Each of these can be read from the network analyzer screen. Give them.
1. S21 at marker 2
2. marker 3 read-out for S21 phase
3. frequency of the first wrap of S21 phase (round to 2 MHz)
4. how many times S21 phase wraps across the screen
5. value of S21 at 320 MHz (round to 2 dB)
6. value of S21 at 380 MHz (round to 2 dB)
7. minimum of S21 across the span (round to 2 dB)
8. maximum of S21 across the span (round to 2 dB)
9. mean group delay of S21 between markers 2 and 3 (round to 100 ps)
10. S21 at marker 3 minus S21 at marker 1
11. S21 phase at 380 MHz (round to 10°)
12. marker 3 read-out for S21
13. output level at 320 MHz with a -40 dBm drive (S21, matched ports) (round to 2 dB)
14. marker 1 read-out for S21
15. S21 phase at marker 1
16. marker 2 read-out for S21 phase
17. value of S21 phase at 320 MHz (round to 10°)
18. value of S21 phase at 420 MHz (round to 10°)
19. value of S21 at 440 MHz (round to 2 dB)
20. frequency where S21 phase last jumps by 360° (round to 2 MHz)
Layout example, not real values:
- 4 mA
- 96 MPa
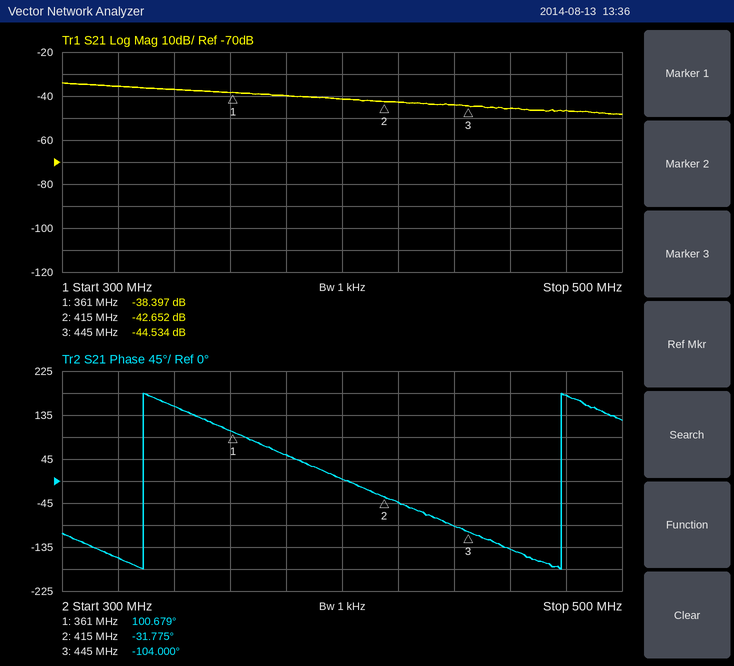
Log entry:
- -42.652 dB
- -104.000°
- 330 MHz
- 2
- -36 dB
- -40 dB
- -48 dB
- -34 dB
- 6.7 ns
- -6.137 dB
- 50°
- -44.534 dB
- -76 dBm
- -38.397 dB
- 100.679°
- -31.775°
- -160°
- -40°
- -44 dB
- 478 MHz
